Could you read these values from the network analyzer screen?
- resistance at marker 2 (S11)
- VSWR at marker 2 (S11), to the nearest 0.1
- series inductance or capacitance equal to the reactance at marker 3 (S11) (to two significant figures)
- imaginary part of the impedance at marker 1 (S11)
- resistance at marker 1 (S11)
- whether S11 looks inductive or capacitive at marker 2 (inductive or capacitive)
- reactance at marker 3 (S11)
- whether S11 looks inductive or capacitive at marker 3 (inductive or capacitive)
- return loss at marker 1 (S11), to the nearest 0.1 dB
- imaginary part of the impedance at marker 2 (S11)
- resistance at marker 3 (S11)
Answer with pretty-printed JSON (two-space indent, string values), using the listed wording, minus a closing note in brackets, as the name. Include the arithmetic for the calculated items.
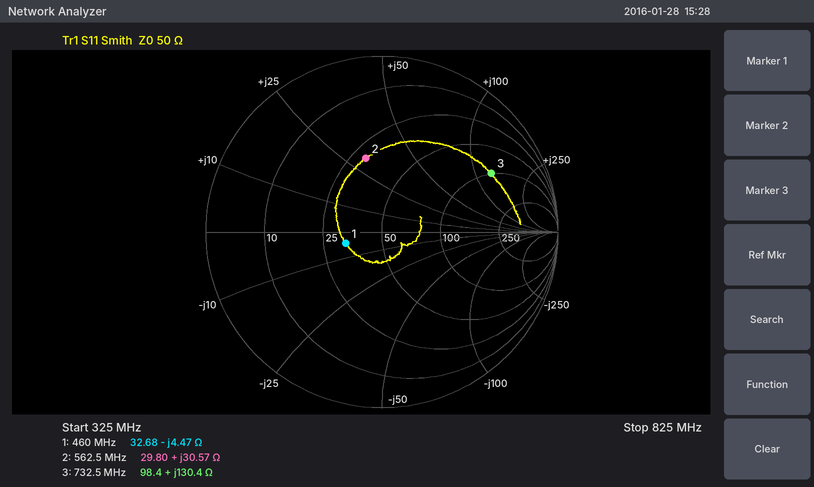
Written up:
{
  "resistance at marker 2": "29.80 Ω",
  "VSWR at marker 2 (S11), to the nearest 0.1": "2.5",
  "series inductance or capacitance equal to the reactance at marker 3 (S11)": "L = 130.4 Ω/(2π × 732.5 MHz) ≈ 28 nH",
  "imaginary part of the impedance at marker 1": "-4.47 Ω",
  "resistance at marker 1": "32.68 Ω",
  "whether S11 looks inductive or capacitive at marker 2": "inductive",
  "reactance at marker 3": "+130.4 Ω",
  "whether S11 looks inductive or capacitive at marker 3": "inductive",
  "return loss at marker 1 (S11), to the nearest 0.1 dB": "13.3 dB",
  "imaginary part of the impedance at marker 2": "+30.57 Ω",
  "resistance at marker 3": "98.4 Ω"
}
